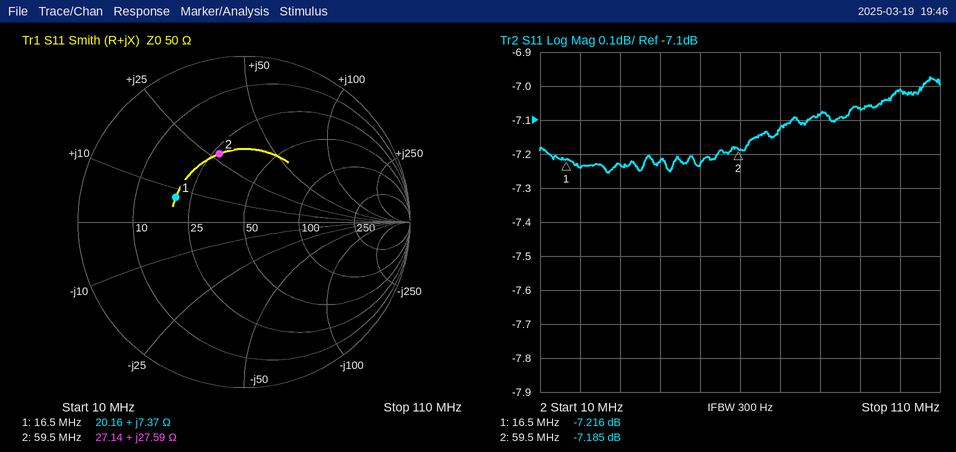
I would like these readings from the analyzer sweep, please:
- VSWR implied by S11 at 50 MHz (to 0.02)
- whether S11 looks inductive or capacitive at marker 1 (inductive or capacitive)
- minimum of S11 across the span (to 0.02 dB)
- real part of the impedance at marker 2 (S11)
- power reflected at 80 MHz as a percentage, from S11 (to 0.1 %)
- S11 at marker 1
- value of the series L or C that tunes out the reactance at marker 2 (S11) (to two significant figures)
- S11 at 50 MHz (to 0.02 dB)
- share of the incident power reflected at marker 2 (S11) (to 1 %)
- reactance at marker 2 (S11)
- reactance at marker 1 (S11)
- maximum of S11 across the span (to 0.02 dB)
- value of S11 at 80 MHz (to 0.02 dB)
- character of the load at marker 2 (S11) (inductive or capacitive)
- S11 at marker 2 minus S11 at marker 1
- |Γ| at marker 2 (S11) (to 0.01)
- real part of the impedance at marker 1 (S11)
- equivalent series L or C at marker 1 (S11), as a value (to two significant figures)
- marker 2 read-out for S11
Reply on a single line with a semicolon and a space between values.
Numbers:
2.54; inductive; -7.26 dB; 27.14 Ω; 19.6 %; -7.216 dB; 97 pF; -7.24 dB; 19 %; +27.59 Ω; +7.37 Ω; -6.98 dB; -7.08 dB; inductive; 0.031 dB; 0.44; 20.16 Ω; 71 nH; -7.185 dB
